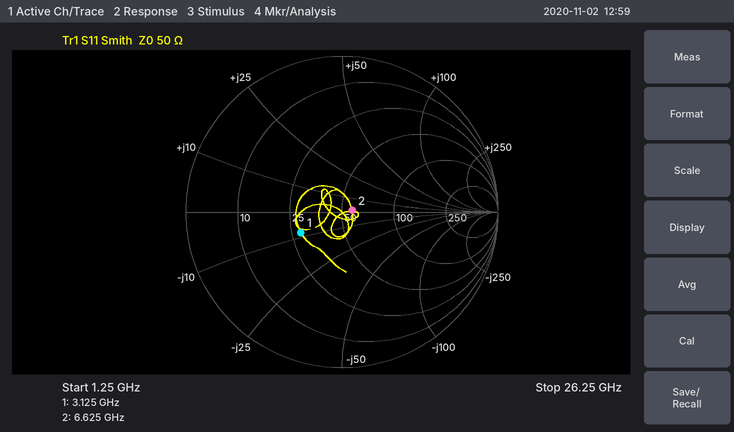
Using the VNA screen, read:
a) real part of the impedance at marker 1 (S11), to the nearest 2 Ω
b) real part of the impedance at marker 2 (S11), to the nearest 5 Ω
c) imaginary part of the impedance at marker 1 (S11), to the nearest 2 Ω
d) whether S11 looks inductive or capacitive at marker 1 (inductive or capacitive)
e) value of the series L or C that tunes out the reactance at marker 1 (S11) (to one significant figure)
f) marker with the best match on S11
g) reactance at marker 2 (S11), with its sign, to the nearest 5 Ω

28 Ω
55 Ω
-8 Ω
capacitive
400 pH
marker 2
0 Ω
